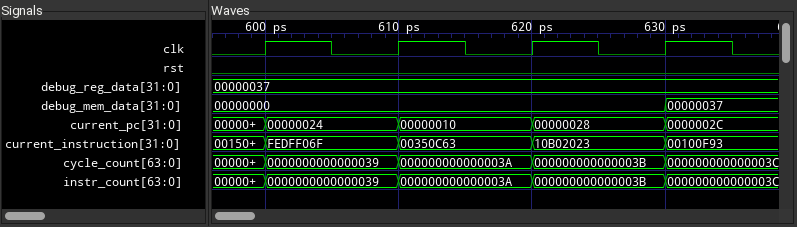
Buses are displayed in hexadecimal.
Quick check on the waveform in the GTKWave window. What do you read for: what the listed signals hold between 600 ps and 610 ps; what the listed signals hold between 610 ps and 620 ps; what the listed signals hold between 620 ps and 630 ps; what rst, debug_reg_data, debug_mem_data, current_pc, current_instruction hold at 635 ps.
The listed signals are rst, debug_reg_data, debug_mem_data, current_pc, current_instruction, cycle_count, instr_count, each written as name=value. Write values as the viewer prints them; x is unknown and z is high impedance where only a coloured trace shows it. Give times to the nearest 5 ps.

rst=0, debug_reg_data=00000037, debug_mem_data=00000000, current_pc=00000024, current_instruction=FEDFF06F, cycle_count=0000000000000039, instr_count=0000000000000039
rst=0, debug_reg_data=00000037, debug_mem_data=00000000, current_pc=00000010, current_instruction=00350C63, cycle_count=000000000000003A, instr_count=000000000000003A
rst=0, debug_reg_data=00000037, debug_mem_data=00000000, current_pc=00000028, current_instruction=10B02023, cycle_count=000000000000003B, instr_count=000000000000003B
rst=0, debug_reg_data=00000037, debug_mem_data=00000037, current_pc=0000002C, current_instruction=00100F93
